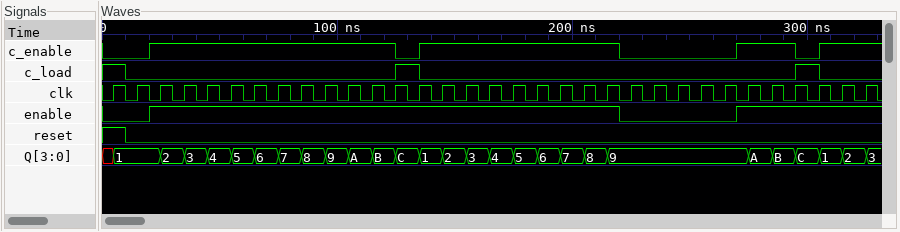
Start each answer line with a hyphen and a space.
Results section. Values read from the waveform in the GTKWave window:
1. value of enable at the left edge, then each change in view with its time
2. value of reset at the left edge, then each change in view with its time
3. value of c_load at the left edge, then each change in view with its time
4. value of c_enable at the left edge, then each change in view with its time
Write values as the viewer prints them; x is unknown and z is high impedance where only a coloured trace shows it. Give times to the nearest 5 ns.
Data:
- 0, 1 at 20 ns, 0 at 220 ns, 1 at 270 ns
- 1, 0 at 10 ns
- 1, 0 at 10 ns, 1 at 125 ns, 0 at 135 ns, 1 at 295 ns, 0 at 305 ns
- 0, 1 at 20 ns, 0 at 125 ns, 1 at 135 ns, 0 at 220 ns, 1 at 270 ns, 0 at 295 ns, 1 at 305 ns
